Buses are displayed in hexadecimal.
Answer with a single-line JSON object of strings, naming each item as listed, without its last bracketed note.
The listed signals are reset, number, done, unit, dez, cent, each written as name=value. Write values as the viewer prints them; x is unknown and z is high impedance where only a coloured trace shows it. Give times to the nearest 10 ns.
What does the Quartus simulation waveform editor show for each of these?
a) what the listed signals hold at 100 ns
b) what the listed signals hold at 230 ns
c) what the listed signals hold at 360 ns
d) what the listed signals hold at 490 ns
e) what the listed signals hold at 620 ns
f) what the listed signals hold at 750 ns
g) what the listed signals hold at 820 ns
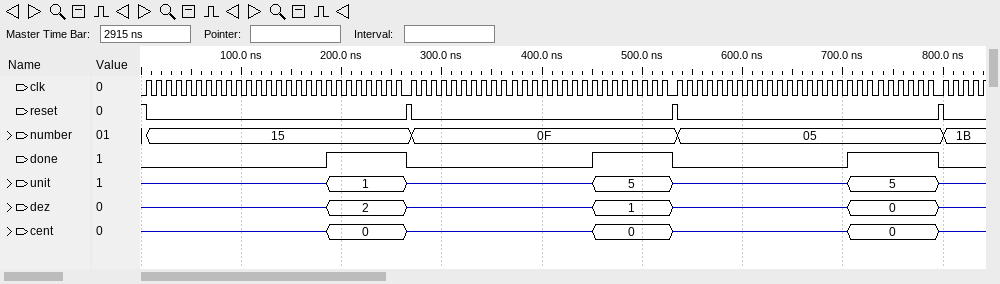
{"what the listed signals hold at 100 ns": "reset=0, number=15, done=0, unit=z, dez=z, cent=z", "what the listed signals hold at 230 ns": "reset=0, number=15, done=1, unit=1, dez=2, cent=0", "what the listed signals hold at 360 ns": "reset=0, number=0F, done=0, unit=z, dez=z, cent=z", "what the listed signals hold at 490 ns": "reset=0, number=0F, done=1, unit=5, dez=1, cent=0", "what the listed signals hold at 620 ns": "reset=0, number=05, done=0, unit=z, dez=z, cent=z", "what the listed signals hold at 750 ns": "reset=0, number=05, done=1, unit=5, dez=0, cent=0", "what the listed signals hold at 820 ns": "reset=0, number=1B, done=0, unit=z, dez=z, cent=z"}
